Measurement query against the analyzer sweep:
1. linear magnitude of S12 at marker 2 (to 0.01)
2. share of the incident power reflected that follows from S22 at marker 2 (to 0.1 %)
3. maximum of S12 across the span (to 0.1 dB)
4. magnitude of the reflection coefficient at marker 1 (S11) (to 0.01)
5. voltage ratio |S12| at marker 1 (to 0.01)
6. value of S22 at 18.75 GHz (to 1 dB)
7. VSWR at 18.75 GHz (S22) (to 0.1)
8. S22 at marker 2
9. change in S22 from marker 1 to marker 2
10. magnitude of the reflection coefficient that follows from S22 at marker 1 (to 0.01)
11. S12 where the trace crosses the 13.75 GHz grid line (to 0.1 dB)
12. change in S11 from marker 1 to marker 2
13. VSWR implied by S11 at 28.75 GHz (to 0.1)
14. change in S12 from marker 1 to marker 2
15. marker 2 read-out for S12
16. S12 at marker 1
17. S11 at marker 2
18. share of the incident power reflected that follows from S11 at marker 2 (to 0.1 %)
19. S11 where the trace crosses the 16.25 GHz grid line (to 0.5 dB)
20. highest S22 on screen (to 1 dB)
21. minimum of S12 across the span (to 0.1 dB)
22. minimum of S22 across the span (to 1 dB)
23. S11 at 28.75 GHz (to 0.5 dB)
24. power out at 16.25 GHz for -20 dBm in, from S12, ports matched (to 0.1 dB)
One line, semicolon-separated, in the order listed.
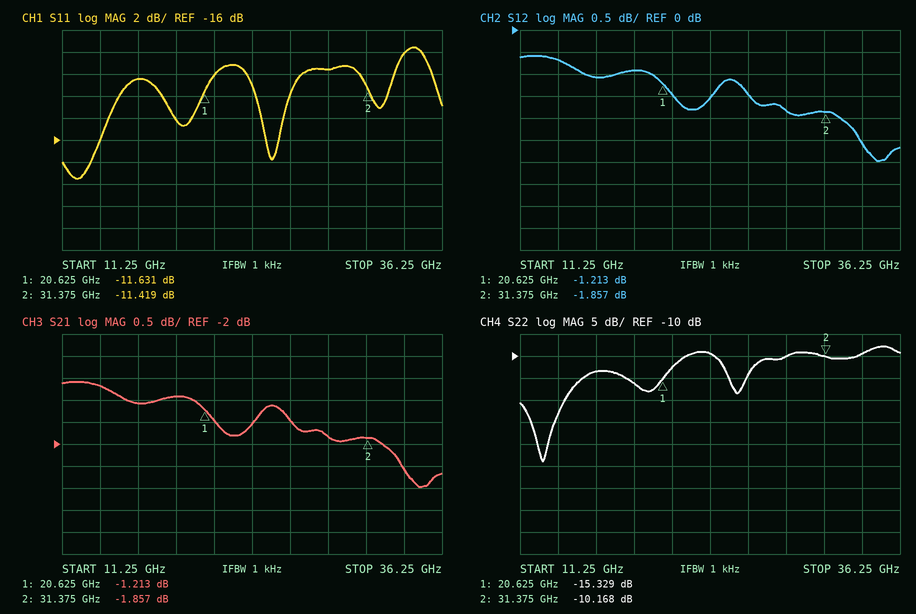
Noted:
0.81; 9.6 %; -0.6 dB; 0.26; 0.87; -16 dB; 1.4; -10.168 dB; 5.161 dB; 0.17; -0.7 dB; 0.212 dB; 2.0; -0.644 dB; -1.857 dB; -1.213 dB; -11.419 dB; 7.2 %; -10.5 dB; -8 dB; -3.0 dB; -34 dB; -9.5 dB; -21.1 dBm
